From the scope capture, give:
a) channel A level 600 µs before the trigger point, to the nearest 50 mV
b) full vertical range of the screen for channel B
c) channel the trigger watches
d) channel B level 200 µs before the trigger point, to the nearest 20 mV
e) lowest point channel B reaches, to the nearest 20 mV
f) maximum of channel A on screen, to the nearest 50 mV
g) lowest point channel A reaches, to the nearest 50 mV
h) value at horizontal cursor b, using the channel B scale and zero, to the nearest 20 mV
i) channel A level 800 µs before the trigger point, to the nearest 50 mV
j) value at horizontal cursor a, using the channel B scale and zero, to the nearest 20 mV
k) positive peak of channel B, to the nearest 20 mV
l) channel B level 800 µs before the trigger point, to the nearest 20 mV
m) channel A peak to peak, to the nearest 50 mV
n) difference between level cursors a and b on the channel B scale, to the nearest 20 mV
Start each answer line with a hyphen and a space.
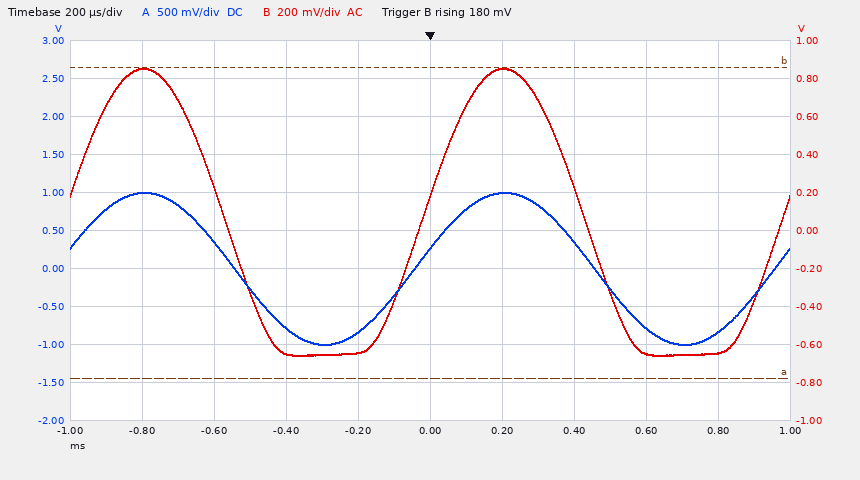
- 350 mV
- 2 V
- channel B
- -640 mV
- -660 mV
- 1.00 V
- -1.00 V
- 860 mV
- 1.00 V
- -780 mV
- 860 mV
- 860 mV
- 2.00 V
- 1.64 V
